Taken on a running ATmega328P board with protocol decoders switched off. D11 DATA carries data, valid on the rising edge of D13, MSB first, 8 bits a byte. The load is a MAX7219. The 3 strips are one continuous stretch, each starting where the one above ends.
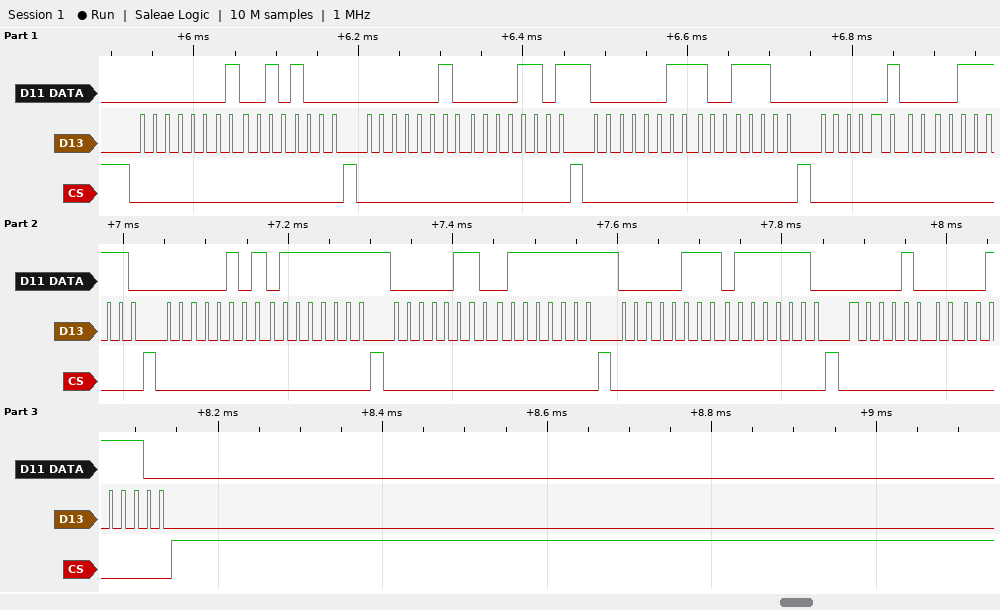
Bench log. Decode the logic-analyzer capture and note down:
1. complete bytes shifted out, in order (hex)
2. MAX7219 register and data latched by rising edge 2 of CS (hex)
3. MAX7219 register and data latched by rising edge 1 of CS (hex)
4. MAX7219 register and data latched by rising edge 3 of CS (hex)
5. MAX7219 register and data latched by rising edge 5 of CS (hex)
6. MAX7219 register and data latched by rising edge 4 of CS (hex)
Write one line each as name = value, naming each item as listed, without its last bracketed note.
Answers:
complete bytes shifted out, in order = 01 28 02 0D 03 9C 04 3E 05 7F 06 7F 07 7E 08 3C
MAX7219 register and data latched by rising edge 2 of CS = register 0x2, data 0x0D
MAX7219 register and data latched by rising edge 1 of CS = register 0x1, data 0x28
MAX7219 register and data latched by rising edge 3 of CS = register 0x3, data 0x9C
MAX7219 register and data latched by rising edge 5 of CS = register 0x5, data 0x7F
MAX7219 register and data latched by rising edge 4 of CS = register 0x4, data 0x3E
